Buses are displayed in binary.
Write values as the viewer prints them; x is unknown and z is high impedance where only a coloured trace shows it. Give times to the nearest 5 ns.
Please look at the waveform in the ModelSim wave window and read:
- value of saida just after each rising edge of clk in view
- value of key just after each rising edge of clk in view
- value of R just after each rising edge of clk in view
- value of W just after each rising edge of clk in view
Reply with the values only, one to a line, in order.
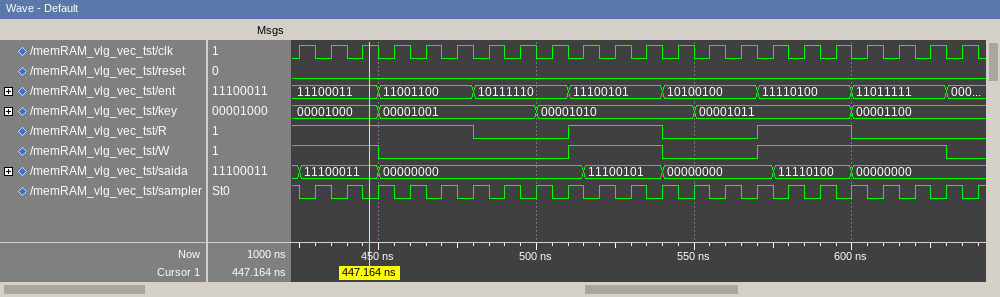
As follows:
11100011, 11100011, 11100011, 00000000, 00000000, 00000000, 00000000, 00000000, 00000000, 11100101, 11100101, 11100101, 00000000, 00000000, 00000000, 11110100, 11110100, 11110100, 00000000, 00000000, 00000000, 00000000
00001000, 00001000, 00001000, 00001001, 00001001, 00001001, 00001001, 00001001, 00001010, 00001010, 00001010, 00001010, 00001010, 00001011, 00001011, 00001011, 00001011, 00001011, 00001100, 00001100, 00001100, 00001100
1 1 1 1 1 1 0 0 0 1 1 1 0 0 0 1 1 1 0 0 0 0
1 1 1 0 0 0 0 0 0 1 1 1 0 0 0 1 1 1 1 1 1 0
